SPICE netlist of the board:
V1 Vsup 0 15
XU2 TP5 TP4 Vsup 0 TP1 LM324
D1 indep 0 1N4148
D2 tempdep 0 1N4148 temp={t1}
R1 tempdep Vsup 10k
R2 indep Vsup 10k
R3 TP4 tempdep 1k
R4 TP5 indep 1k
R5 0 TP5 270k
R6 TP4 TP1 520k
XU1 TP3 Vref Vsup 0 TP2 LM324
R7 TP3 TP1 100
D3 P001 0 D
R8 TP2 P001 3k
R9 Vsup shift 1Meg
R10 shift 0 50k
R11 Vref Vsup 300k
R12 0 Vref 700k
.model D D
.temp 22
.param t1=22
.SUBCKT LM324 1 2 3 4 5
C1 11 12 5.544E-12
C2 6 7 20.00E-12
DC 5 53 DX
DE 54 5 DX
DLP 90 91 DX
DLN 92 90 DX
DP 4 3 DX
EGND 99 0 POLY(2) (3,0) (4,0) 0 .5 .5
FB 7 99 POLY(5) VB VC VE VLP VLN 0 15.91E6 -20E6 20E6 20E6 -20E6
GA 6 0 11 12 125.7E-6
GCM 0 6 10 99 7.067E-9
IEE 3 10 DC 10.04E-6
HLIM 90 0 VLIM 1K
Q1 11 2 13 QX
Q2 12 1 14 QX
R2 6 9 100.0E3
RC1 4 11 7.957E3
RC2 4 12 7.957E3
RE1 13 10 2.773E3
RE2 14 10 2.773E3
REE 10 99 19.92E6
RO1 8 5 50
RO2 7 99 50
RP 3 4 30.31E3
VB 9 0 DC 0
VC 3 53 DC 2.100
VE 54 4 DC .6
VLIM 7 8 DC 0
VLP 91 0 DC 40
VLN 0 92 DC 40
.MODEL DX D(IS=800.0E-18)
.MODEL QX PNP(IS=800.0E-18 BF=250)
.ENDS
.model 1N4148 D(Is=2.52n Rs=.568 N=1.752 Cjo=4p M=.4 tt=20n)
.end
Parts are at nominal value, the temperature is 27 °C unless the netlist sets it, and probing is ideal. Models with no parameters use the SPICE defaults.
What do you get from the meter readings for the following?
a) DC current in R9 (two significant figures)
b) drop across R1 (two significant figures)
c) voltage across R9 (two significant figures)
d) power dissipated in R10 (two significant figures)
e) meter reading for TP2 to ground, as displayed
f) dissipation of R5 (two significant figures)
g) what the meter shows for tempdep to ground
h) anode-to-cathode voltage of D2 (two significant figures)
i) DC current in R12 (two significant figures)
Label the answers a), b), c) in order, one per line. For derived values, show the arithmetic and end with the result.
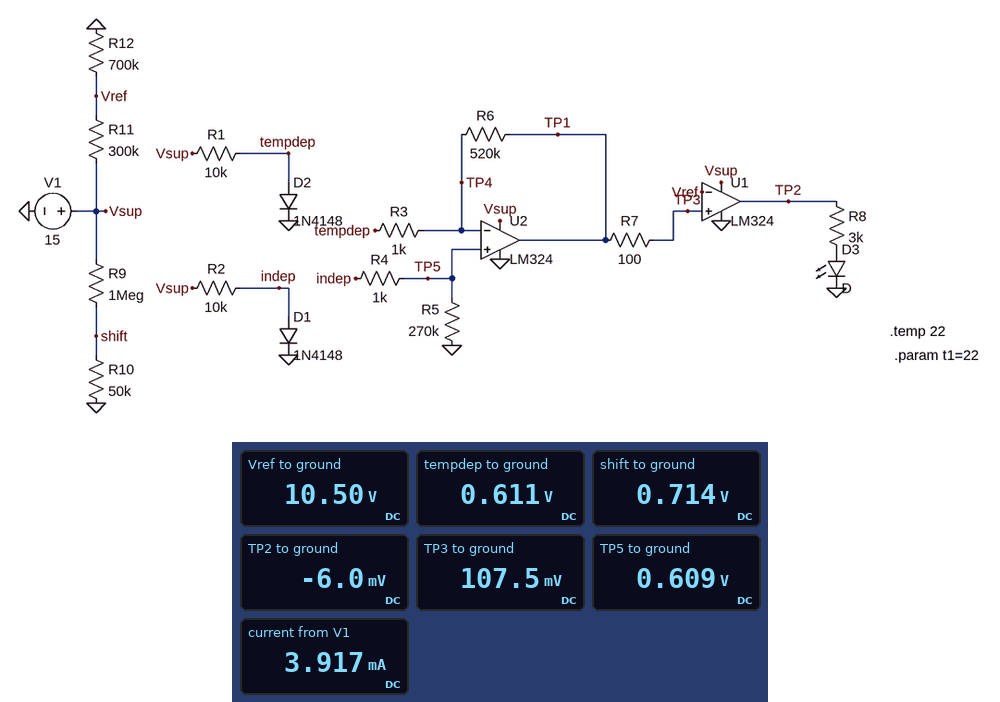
a) (15 V - 714 mV) / 1 MΩ = 14 µA
b) 15 V - 611 mV = 14 V
c) 15 V - 714 mV = 14 V
d) (714 mV)^2 / 50 kΩ = 10 µW
e) -6.0 mV
f) (609 mV)^2 / 270 kΩ = 1.4 µW
g) 0.611 V
h) 611 mV = 610 mV
i) (10.5 V) / 700 kΩ = 15 µA
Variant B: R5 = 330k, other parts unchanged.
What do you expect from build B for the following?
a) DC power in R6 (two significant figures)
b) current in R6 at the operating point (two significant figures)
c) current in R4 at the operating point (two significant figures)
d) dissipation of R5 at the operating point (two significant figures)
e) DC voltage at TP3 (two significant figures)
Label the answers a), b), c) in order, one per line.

a) 460 nW
b) 940 nA
c) 1.8 µA
d) 1.1 µW
e) 120 mV
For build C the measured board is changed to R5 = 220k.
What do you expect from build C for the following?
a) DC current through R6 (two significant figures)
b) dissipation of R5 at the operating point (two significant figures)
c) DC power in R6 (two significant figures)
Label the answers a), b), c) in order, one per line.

a) 990 nA
b) 1.7 µW
c) 510 nW
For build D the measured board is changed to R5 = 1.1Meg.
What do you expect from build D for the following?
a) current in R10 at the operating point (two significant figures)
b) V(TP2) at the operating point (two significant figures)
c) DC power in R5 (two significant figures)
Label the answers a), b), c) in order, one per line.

a) 14 µA
b) -5.9 mV
c) 340 nW
